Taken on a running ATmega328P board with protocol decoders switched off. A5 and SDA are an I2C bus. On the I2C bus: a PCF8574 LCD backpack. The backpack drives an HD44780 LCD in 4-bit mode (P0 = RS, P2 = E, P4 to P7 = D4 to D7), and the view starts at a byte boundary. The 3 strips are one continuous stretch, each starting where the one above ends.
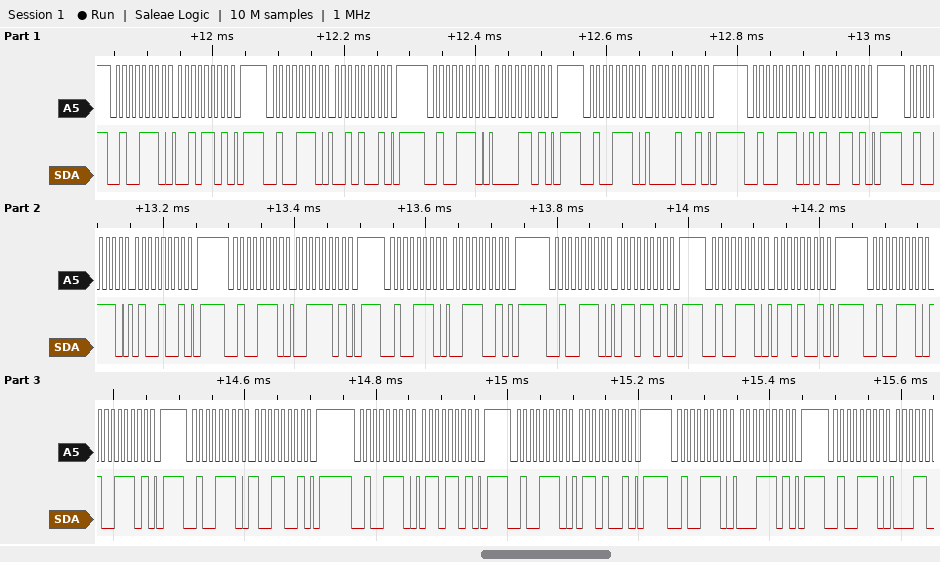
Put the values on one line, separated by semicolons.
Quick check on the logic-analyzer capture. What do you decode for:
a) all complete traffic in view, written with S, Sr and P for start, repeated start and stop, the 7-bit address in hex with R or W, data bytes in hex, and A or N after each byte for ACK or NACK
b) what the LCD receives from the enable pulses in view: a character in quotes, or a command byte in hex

S 27W A 2D A P S 27W A 29 A P S 27W A 0D A P S 27W A 09 A P S 27W A 4D A P S 27W A 49 A P S 27W A 3D A P S 27W A 39 A P S 27W A 6D A P S 27W A 69 A P S 27W A 9D A P S 27W A 99 A P S 27W A 6D A P S 27W A 69 A P S 27W A 1D A P S 27W A; ' ' 'C' 'i'
